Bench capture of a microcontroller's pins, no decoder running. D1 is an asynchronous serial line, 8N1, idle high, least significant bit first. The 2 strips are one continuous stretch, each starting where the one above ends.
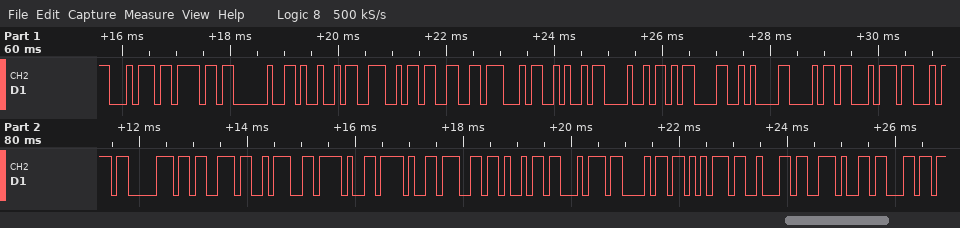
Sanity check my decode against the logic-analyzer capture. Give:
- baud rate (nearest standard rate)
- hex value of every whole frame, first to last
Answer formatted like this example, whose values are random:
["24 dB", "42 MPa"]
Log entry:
["9600 baud", "74 6F 20 49 4E 33 47 4A 48 0D 0A 68 74 74 70 73 3A 2F 2F 67 69 74 68 75 62 2E 63"]
